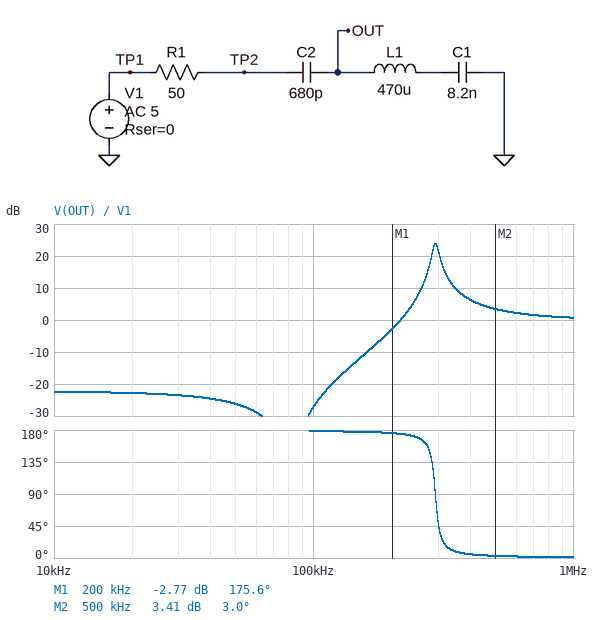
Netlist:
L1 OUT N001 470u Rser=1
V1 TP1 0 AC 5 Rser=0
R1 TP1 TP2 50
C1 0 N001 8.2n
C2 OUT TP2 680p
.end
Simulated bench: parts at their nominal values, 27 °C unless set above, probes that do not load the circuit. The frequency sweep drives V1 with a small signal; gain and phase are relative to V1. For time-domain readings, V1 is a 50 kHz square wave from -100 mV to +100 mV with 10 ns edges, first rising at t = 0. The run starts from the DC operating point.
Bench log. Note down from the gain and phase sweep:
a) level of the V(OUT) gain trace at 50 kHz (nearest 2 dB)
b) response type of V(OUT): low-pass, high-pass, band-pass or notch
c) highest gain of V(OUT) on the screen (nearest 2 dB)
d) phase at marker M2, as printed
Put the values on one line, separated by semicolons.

-26 dB; band-pass; 24 dB; 3.0 deg
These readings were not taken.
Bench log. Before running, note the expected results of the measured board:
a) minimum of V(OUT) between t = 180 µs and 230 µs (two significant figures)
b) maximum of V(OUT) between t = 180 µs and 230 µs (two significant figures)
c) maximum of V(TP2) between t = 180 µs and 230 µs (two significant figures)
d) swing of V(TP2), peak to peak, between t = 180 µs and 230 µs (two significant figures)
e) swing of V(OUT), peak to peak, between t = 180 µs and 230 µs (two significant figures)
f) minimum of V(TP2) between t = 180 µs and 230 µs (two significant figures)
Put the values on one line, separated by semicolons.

-120 mV; 130 mV; 110 mV; 210 mV; 250 mV; -110 mV
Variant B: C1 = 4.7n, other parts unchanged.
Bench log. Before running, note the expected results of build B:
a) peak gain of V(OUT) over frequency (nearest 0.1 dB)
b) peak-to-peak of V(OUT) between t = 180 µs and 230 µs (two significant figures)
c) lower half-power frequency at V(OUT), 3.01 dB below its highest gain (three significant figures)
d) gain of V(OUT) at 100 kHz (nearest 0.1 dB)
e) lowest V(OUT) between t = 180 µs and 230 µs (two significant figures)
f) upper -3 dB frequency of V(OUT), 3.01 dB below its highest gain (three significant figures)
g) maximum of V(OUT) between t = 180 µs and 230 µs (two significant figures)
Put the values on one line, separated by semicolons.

23.7 dB; 250 mV; 293 kHz; -34.8 dB; -110 mV; 311 kHz; 140 mV
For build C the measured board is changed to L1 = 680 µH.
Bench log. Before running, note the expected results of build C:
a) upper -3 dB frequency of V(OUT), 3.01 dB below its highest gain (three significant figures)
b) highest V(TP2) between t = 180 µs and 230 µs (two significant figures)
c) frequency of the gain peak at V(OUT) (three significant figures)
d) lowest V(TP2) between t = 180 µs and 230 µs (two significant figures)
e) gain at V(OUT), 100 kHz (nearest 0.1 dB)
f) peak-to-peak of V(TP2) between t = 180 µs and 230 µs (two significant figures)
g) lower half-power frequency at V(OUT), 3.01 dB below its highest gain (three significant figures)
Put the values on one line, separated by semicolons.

250 kHz; 120 mV; 244 kHz; -120 mV; -19.1 dB; 240 mV; 238 kHz
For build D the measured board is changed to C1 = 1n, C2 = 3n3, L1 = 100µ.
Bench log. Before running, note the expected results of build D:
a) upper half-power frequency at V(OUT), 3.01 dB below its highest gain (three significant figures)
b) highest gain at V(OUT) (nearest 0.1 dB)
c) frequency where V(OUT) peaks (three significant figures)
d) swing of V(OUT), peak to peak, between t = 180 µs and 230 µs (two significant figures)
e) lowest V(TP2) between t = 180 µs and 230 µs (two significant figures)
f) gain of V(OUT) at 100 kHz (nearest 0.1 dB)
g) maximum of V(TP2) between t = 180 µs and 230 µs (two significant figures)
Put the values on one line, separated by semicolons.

731 kHz; 5.4 dB; 597 kHz; 240 mV; -120 mV; -2.4 dB; 120 mV
